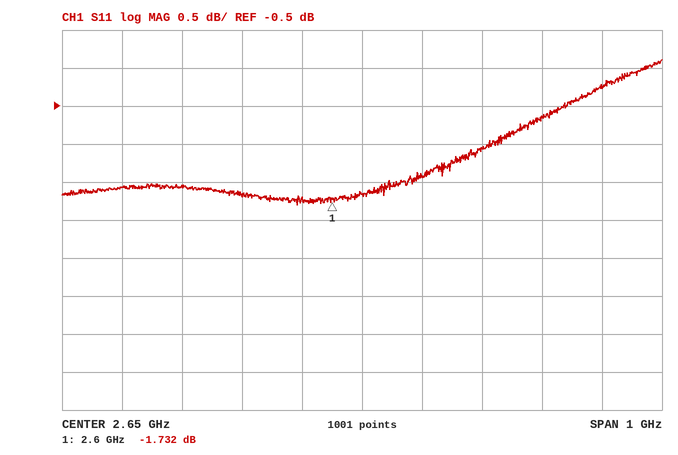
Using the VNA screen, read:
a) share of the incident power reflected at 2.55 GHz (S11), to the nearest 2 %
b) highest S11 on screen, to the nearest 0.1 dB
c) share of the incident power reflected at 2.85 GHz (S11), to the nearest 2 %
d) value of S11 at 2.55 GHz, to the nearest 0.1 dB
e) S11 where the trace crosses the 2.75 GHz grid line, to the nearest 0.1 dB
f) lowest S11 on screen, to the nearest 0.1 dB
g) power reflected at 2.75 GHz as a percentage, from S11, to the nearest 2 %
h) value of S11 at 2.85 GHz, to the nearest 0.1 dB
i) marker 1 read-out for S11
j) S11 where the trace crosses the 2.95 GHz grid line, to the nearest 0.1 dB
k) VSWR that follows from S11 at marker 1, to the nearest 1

68 %
0.1 dB
78 %
-1.7 dB
-1.4 dB
-1.8 dB
72 %
-1.1 dB
-1.732 dB
-0.6 dB
10
